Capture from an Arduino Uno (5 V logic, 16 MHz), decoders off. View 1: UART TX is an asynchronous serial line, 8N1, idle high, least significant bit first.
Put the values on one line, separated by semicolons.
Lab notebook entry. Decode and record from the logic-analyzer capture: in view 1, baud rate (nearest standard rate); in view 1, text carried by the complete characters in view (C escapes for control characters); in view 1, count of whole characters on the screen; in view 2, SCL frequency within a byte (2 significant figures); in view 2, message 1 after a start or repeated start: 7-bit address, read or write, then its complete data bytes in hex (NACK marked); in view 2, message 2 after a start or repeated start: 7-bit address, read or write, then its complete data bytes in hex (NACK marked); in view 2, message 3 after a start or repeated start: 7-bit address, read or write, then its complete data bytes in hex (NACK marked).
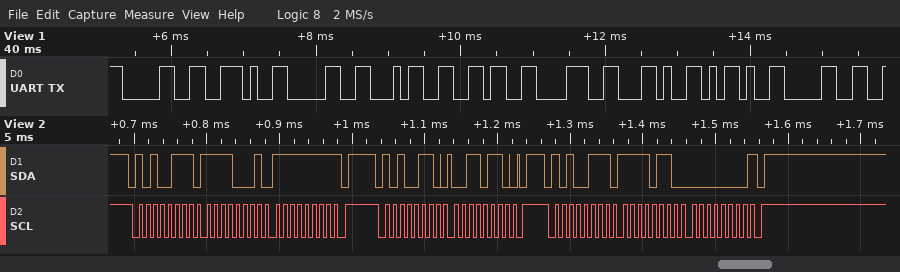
9600 baud; "0.0468,-0"; 9; 100 kHz; 0x53 read: F1 FF NACK; 0x53 write: 36; 0x53 read: F6 00 NACK
